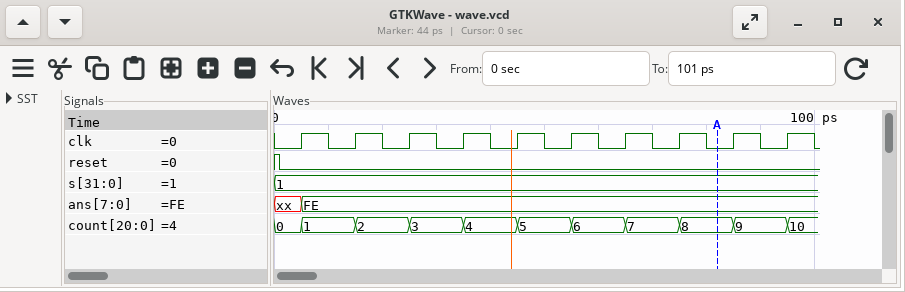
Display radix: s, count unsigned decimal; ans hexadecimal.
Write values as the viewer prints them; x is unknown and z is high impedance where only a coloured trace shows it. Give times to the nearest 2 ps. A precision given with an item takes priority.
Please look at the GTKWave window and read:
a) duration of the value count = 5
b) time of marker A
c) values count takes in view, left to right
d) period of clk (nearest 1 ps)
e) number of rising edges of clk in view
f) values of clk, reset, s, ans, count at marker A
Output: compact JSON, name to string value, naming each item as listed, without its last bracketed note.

{"duration of the value count = 5": "10 ps", "time of marker A": "82 ps", "values count takes in view, left to right": "0, 1, 2, 3, 4, 5, 6, 7, 8, 9, 10", "period of clk": "10 ps", "number of rising edges of clk in view": "10", "values of clk, reset, s, ans, count at marker A": "clk=0, reset=0, s=1, ans=FE, count=8"}
